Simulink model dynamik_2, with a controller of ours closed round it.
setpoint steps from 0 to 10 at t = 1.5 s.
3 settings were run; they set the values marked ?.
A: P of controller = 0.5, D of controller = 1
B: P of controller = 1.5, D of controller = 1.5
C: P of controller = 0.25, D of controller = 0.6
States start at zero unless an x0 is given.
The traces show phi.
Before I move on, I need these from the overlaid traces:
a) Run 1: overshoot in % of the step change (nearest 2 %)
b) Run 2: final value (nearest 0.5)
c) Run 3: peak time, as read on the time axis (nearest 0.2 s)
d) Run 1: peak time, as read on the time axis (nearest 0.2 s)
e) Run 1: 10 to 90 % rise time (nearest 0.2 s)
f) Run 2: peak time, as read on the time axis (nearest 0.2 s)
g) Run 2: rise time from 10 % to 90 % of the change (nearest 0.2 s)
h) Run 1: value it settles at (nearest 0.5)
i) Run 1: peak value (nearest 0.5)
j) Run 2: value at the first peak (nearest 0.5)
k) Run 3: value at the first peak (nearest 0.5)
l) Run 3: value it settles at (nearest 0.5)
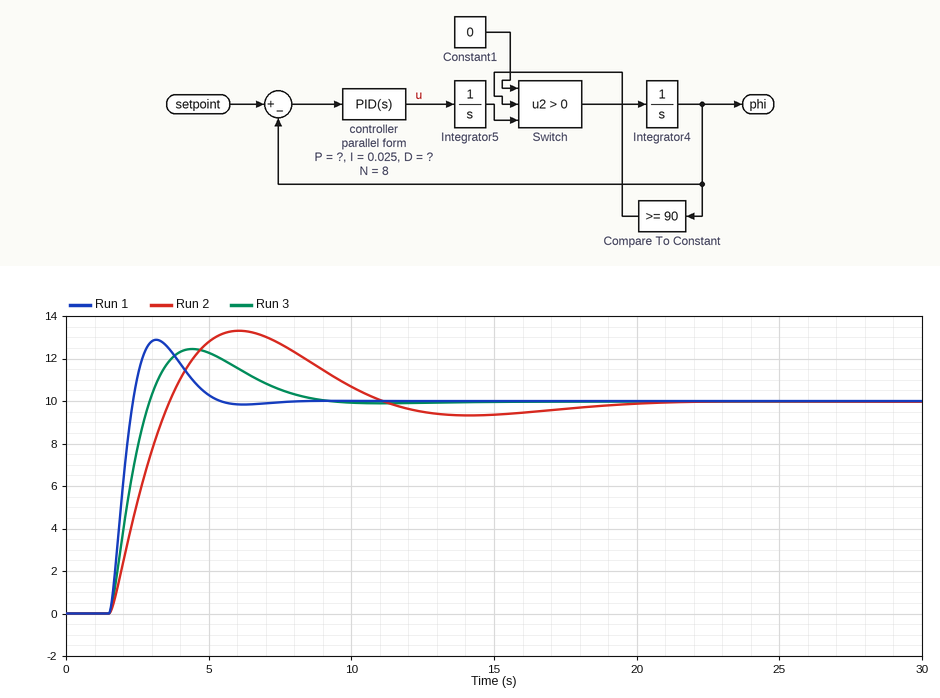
28 %
10.0
4.4 s
3.2 s
0.6 s
6.0 s
1.6 s
10.0
13.0
13.5
12.5
10.0
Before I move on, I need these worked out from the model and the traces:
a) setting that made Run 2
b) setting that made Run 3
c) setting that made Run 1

C
A
B
